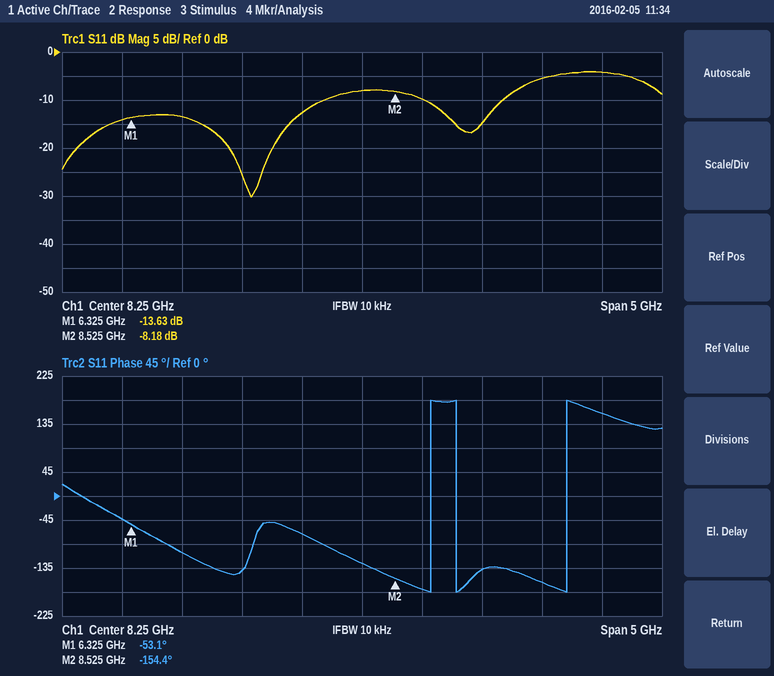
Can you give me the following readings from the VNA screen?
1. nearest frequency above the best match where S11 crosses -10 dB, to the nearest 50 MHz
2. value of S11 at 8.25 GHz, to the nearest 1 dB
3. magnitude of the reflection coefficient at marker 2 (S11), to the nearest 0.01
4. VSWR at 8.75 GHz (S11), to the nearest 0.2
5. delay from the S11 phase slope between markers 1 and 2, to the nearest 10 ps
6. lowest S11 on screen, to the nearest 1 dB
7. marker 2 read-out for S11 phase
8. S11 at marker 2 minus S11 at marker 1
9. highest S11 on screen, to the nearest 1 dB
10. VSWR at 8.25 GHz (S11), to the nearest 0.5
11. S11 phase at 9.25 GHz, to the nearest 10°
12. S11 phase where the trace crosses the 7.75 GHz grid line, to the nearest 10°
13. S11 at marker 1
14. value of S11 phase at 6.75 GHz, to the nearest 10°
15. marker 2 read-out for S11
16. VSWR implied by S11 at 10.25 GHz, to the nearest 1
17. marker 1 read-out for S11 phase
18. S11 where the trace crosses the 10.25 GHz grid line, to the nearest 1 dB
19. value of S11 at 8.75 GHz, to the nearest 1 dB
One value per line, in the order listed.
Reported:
7.95 GHz
-8 dB
0.39
2.0
130 ps
-30 dB
-154.4°
5.45 dB
-4 dB
2.5
-140°
-70°
-13.63 dB
-110°
-8.18 dB
4
-53.1°
-4 dB
-10 dB
